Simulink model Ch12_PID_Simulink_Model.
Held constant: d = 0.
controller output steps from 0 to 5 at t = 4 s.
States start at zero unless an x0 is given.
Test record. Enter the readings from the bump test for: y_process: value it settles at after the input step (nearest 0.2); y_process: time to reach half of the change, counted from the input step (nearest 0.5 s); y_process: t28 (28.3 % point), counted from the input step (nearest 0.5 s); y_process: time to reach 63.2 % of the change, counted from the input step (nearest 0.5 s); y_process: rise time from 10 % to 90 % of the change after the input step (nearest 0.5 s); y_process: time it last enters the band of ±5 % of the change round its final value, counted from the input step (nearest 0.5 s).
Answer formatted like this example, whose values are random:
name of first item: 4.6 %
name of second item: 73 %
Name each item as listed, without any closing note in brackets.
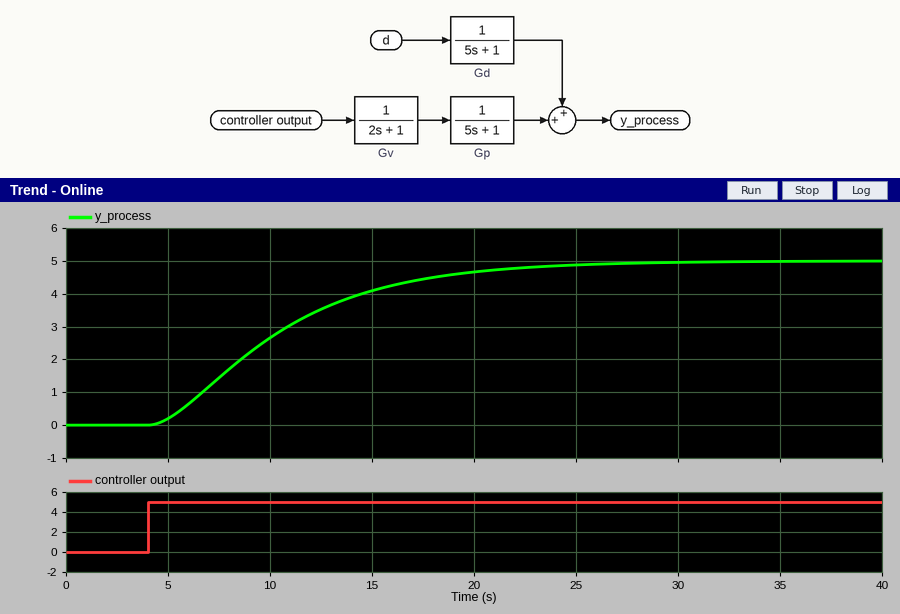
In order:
y_process: value it settles at after the input step: 5.0
y_process: time to reach half of the change, counted from the input step: 5.5 s
y_process: t28 (28.3 % point), counted from the input step: 3.5 s
y_process: time to reach 63.2 % of the change, counted from the input step: 7.5 s
y_process: rise time from 10 % to 90 % of the change after the input step: 12.5 s
y_process: time it last enters the band of ±5 % of the change round its final value, counted from the input step: 17.5 s
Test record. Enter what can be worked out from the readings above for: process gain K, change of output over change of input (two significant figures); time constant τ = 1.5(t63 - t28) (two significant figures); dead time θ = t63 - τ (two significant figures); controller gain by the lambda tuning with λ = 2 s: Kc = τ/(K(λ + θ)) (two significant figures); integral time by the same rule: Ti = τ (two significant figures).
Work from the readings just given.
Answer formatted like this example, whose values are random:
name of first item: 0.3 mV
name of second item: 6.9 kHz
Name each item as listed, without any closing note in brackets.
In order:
process gain K, change of output over change of input: 1.0
time constant τ = 1.5(t63 - t28): 6.0 s
dead time θ = t63 - τ: 1.5 s
controller gain by the lambda tuning with λ = 2 s: Kc = τ/(K(λ + θ)): 1.7
integral time by the same rule: Ti = τ: 6.0 s
